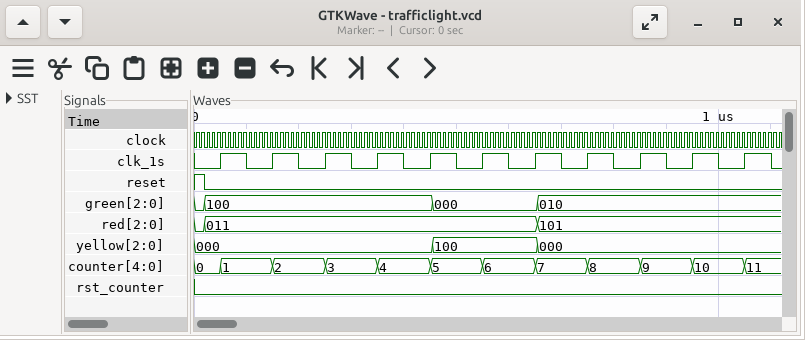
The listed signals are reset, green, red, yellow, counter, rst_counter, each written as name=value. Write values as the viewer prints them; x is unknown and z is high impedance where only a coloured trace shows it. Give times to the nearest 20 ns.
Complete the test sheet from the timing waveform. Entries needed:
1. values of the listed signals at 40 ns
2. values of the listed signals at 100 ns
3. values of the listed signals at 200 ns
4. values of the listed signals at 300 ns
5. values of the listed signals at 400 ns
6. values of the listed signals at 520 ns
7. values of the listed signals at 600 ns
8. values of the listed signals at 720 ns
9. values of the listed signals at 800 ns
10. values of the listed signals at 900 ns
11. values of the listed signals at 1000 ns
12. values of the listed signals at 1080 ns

reset=0, green=100, red=011, yellow=000, counter=0, rst_counter=0
reset=0, green=100, red=011, yellow=000, counter=1, rst_counter=0
reset=0, green=100, red=011, yellow=000, counter=2, rst_counter=0
reset=0, green=100, red=011, yellow=000, counter=3, rst_counter=0
reset=0, green=100, red=011, yellow=000, counter=4, rst_counter=0
reset=0, green=000, red=011, yellow=100, counter=5, rst_counter=0
reset=0, green=000, red=011, yellow=100, counter=6, rst_counter=0
reset=0, green=010, red=101, yellow=000, counter=7, rst_counter=0
reset=0, green=010, red=101, yellow=000, counter=8, rst_counter=0
reset=0, green=010, red=101, yellow=000, counter=9, rst_counter=0
reset=0, green=010, red=101, yellow=000, counter=10, rst_counter=0
reset=0, green=010, red=101, yellow=000, counter=11, rst_counter=0
